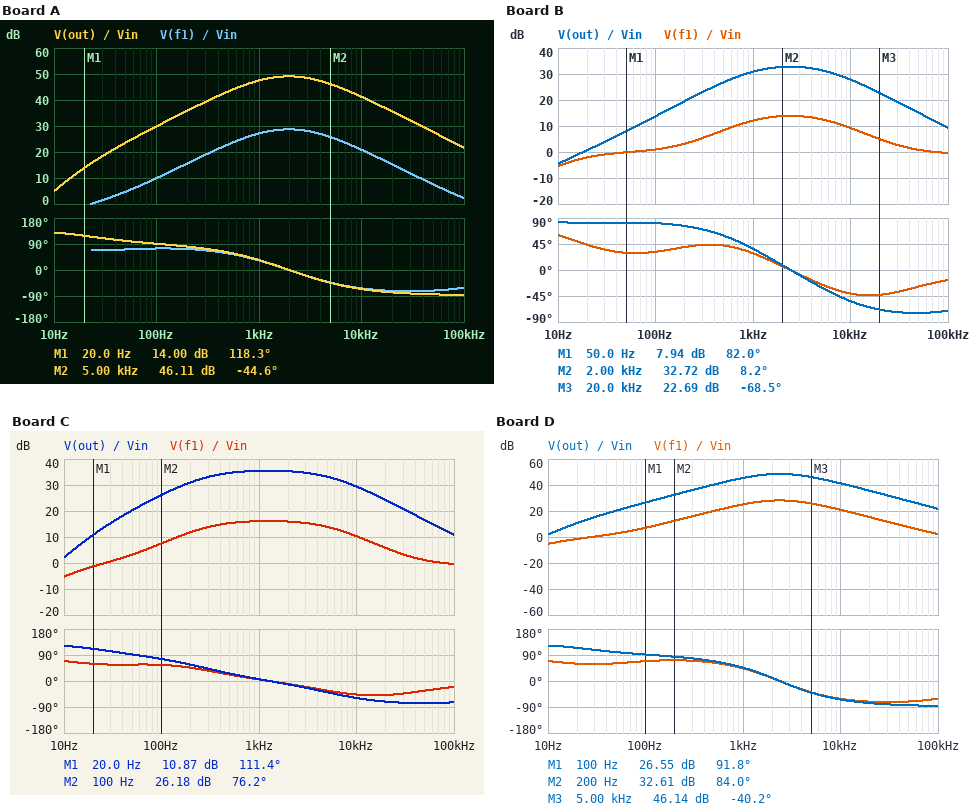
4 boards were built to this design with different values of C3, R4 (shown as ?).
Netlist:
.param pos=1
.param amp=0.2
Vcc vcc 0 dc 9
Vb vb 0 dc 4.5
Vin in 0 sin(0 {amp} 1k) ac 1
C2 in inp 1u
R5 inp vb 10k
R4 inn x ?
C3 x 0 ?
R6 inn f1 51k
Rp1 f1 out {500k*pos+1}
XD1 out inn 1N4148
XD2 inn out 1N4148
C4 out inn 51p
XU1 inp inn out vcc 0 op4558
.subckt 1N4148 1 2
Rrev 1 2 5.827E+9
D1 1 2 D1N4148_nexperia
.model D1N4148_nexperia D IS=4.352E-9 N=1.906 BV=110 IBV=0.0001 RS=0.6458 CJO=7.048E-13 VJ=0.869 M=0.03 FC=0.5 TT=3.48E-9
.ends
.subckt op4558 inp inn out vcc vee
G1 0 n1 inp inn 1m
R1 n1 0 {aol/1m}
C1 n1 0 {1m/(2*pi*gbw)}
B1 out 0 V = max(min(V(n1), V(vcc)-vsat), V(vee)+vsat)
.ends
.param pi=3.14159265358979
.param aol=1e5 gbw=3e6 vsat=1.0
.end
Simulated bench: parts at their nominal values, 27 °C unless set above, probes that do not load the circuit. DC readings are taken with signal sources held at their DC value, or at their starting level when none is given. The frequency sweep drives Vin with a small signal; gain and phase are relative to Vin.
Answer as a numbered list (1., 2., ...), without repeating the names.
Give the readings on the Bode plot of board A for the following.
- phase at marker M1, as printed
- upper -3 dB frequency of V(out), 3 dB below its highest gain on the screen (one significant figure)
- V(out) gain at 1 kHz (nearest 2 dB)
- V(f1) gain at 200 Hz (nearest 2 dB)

1. 118.3 deg
2. 5 kHz
3. 48 dB
4. 16 dB
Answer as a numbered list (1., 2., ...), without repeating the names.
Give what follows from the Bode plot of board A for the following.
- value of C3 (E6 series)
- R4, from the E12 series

1. 100 nF
2. 1.5 kΩ
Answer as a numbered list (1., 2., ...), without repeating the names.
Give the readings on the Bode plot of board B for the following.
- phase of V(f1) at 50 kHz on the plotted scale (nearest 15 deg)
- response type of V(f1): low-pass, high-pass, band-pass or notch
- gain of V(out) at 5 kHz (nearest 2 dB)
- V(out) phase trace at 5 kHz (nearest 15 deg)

1. -30 deg
2. band-pass
3. 32 dB
4. -30 deg
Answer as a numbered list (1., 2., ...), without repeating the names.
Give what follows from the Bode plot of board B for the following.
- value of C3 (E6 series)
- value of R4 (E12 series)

1. 15 nF
2. 10 kΩ
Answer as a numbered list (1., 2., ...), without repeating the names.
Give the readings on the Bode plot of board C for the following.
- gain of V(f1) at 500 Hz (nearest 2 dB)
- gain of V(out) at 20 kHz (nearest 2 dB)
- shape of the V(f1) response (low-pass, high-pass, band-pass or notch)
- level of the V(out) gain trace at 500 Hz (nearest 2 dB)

1. 16 dB
2. 24 dB
3. band-pass
4. 34 dB
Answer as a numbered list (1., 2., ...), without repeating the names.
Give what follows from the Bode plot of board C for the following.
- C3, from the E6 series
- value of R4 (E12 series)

1. 68 nF
2. 8.2 kΩ
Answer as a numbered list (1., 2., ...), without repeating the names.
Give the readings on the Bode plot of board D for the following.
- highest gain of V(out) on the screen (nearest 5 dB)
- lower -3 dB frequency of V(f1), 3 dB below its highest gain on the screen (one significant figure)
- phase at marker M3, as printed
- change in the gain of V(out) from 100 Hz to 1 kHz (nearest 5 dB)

1. 50 dB
2. 1 kHz
3. -40.2 deg
4. 20 dB
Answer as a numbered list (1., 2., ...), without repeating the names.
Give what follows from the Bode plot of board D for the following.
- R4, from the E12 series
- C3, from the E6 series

1. 1.5 kΩ
2. 68 nF
